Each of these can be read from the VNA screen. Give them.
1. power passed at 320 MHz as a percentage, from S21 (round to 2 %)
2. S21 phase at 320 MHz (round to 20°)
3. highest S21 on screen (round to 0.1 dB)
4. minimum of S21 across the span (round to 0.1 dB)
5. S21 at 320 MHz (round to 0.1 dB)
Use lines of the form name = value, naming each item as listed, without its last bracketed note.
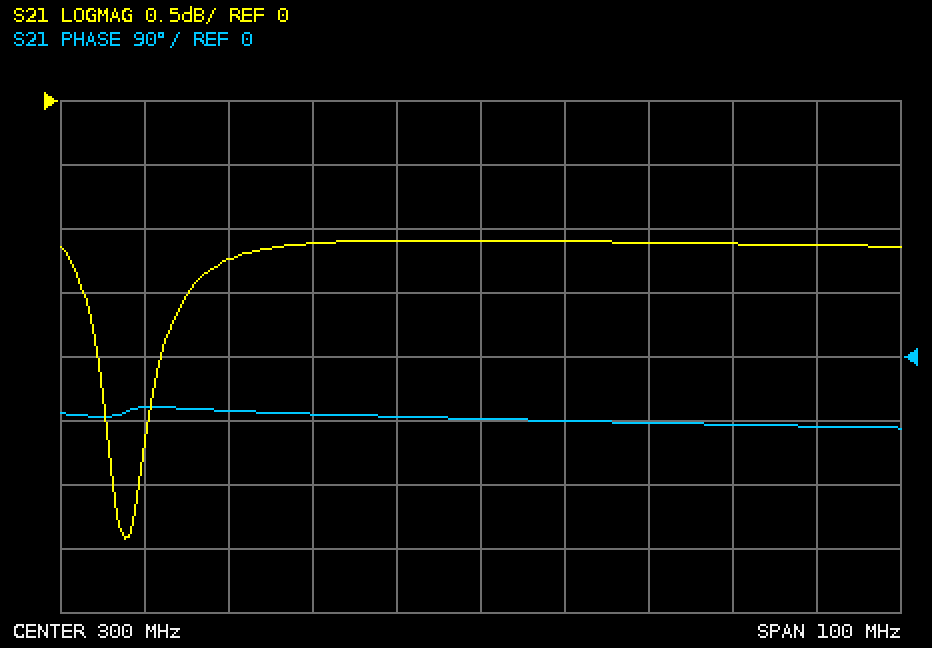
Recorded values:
power passed at 320 MHz as a percentage, from S21 = 78 %
S21 phase at 320 MHz = -100°
highest S21 on screen = -1.1 dB
minimum of S21 across the span = -3.4 dB
S21 at 320 MHz = -1.1 dB
